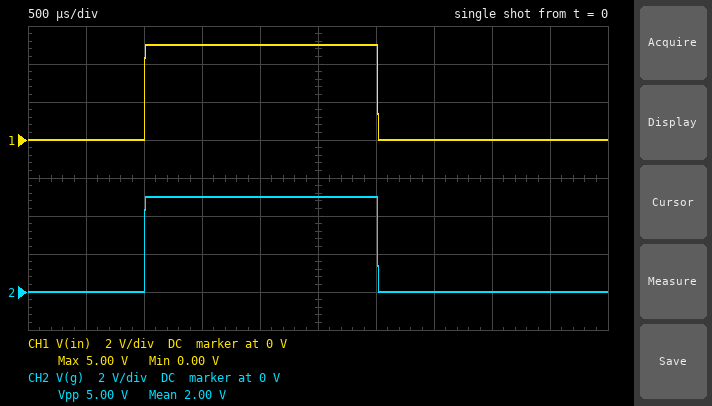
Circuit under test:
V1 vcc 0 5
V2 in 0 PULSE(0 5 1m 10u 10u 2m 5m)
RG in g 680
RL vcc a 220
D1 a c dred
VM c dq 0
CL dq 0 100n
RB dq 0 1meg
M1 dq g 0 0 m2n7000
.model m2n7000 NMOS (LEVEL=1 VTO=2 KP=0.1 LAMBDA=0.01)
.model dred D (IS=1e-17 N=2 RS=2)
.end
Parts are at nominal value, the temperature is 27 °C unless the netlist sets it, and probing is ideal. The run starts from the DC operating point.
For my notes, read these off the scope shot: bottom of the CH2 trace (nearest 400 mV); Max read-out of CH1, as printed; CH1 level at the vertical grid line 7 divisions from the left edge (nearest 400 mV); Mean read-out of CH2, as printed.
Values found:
0 V
5.00 V
0 V
2.00 V
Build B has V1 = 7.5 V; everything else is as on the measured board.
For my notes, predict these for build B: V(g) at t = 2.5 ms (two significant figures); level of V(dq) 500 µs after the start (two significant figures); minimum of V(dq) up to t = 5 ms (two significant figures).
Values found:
5.0 V
6.1 V
85 mV
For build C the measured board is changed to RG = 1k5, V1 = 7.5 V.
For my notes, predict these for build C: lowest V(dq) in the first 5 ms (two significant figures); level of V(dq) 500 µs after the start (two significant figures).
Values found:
85 mV
6.1 V
